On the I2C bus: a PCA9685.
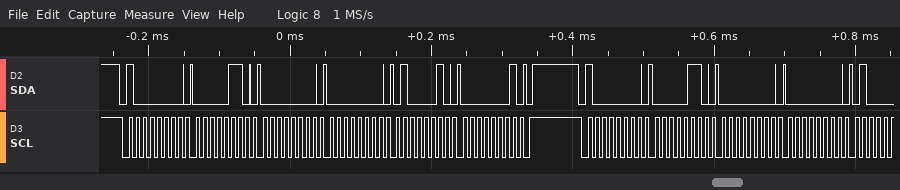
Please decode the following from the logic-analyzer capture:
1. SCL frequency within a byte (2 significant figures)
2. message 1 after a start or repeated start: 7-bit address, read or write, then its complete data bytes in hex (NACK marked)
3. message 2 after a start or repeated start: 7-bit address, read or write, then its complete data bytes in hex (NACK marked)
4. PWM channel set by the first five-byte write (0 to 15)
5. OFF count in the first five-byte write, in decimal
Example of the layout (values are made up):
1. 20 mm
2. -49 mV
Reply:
1. 100 kHz
2. 0x40 write: 06 00 00 42 01
3. 0x40 write: 06 00 00
4. 0
5. 322
